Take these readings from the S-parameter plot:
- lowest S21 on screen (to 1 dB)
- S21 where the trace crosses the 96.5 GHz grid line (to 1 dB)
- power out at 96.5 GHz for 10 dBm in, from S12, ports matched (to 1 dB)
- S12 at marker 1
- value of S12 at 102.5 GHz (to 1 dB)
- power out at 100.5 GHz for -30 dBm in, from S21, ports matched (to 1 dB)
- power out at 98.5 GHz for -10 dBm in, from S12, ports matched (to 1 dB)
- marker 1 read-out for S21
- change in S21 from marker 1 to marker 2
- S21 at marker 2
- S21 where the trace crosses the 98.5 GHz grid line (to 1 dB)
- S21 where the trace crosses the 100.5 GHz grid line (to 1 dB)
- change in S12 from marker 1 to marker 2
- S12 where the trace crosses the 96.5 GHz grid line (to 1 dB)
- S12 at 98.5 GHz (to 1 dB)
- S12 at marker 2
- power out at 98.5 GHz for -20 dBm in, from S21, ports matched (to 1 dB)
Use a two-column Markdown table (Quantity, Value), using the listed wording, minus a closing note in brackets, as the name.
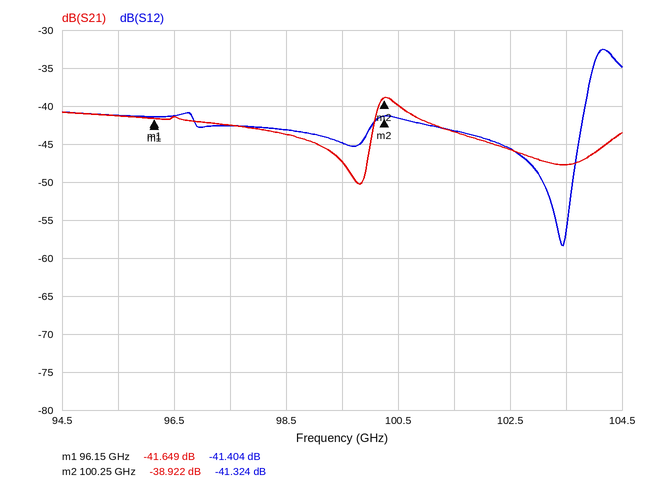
| Quantity | Value |
|---|---|
| lowest S21 on screen | -50 dB |
| S21 where the trace crosses the 96.5 GHz grid line | -41 dB |
| power out at 96.5 GHz for 10 dBm in, from S12, ports matched | -31 dBm |
| S12 at marker 1 | -41.404 dB |
| value of S12 at 102.5 GHz | -46 dB |
| power out at 100.5 GHz for -30 dBm in, from S21, ports matched | -70 dBm |
| power out at 98.5 GHz for -10 dBm in, from S12, ports matched | -53 dBm |
| marker 1 read-out for S21 | -41.649 dB |
| change in S21 from marker 1 to marker 2 | 2.727 dB |
| S21 at marker 2 | -38.922 dB |
| S21 where the trace crosses the 98.5 GHz grid line | -44 dB |
| S21 where the trace crosses the 100.5 GHz grid line | -40 dB |
| change in S12 from marker 1 to marker 2 | 0.080 dB |
| S12 where the trace crosses the 96.5 GHz grid line | -41 dB |
| S12 at 98.5 GHz | -43 dB |
| S12 at marker 2 | -41.324 dB |
| power out at 98.5 GHz for -20 dBm in, from S21, ports matched | -64 dBm |
